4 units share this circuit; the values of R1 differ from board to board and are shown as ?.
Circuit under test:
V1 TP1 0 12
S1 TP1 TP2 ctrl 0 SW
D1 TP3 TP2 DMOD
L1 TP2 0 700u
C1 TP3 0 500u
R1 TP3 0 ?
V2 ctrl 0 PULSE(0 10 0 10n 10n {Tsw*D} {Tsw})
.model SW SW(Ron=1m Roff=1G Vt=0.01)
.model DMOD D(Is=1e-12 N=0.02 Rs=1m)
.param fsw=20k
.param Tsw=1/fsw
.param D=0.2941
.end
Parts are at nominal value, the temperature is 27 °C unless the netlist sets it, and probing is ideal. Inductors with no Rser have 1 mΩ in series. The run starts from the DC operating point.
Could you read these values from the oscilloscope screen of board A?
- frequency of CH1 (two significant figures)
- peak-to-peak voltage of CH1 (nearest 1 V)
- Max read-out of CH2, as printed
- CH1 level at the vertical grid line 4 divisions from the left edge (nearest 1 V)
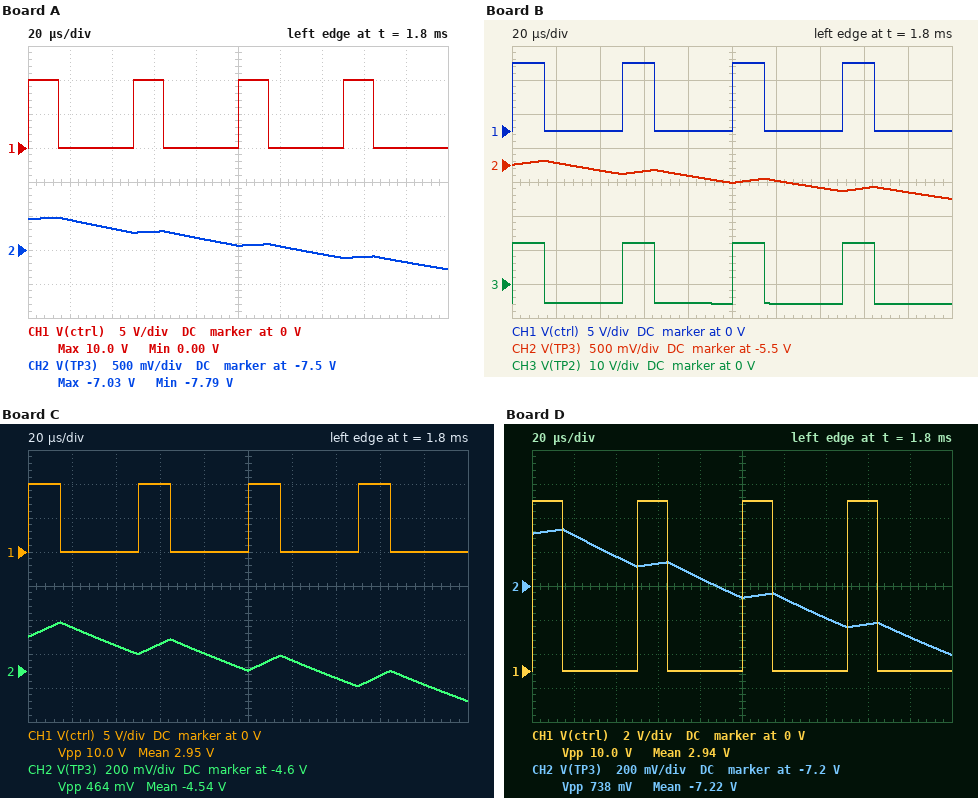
20 kHz
10 V
-7.03 V
0 V
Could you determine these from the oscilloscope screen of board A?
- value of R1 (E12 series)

10 Ω
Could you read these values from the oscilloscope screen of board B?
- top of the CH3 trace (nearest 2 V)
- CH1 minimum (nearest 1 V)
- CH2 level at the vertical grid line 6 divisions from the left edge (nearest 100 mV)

12 V
0 V
-5.7 V
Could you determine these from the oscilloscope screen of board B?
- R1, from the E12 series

2.7 Ω
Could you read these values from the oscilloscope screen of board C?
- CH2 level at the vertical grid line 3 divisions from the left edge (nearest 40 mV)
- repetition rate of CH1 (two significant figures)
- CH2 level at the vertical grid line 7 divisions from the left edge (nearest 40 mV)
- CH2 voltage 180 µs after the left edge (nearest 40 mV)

-4.44 V
20 kHz
-4.64 V
-4.68 V
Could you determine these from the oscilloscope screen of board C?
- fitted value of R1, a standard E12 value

1.5 Ω
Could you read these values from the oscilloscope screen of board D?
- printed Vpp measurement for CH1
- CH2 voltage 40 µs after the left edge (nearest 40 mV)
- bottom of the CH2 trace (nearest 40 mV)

10.0 V
-7.04 V
-7.60 V
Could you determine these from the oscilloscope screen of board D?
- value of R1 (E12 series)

8.2 Ω
